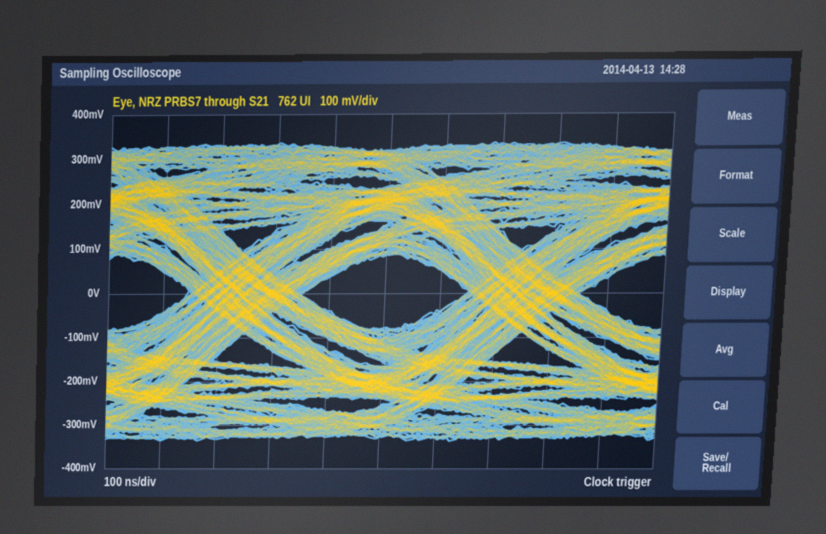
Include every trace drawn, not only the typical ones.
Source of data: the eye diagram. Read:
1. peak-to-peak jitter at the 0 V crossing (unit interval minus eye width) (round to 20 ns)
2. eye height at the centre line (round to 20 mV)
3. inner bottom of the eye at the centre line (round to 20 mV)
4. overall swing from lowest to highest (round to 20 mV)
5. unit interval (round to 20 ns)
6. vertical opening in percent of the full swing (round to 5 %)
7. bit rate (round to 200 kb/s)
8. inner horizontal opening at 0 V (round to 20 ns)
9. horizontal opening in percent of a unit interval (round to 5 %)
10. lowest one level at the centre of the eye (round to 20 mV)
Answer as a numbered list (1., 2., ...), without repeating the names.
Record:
1. 200 ns
2. 160 mV
3. -80 mV
4. 680 mV
5. 500 ns
6. 25 %
7. 2.0 Mb/s
8. 300 ns
9. 60 %
10. 80 mV
